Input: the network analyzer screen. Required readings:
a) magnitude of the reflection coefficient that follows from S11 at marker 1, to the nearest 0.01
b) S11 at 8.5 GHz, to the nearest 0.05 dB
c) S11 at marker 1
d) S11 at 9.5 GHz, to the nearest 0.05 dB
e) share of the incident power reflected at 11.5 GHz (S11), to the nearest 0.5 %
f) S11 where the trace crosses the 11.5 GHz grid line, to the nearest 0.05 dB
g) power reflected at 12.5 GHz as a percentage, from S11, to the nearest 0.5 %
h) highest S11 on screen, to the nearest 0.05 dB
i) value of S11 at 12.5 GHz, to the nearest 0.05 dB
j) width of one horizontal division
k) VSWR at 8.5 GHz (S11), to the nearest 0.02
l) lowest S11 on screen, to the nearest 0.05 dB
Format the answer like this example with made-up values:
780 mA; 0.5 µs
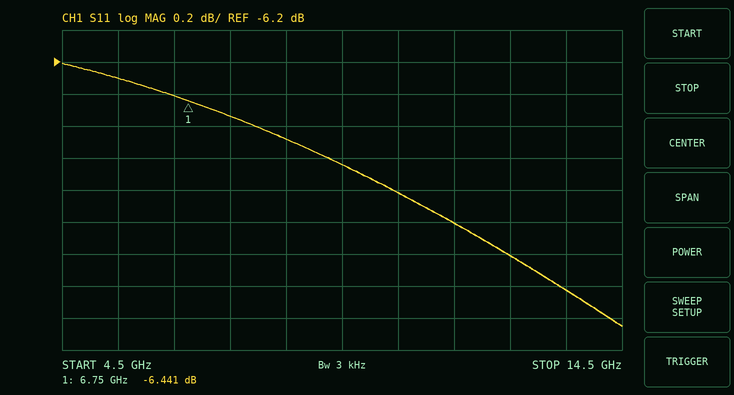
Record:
0.48; -6.70 dB; -6.441 dB; -6.85 dB; 19.0 %; -7.20 dB; 18.0 %; -6.20 dB; -7.40 dB; 1 GHz; 2.72; -7.85 dB
